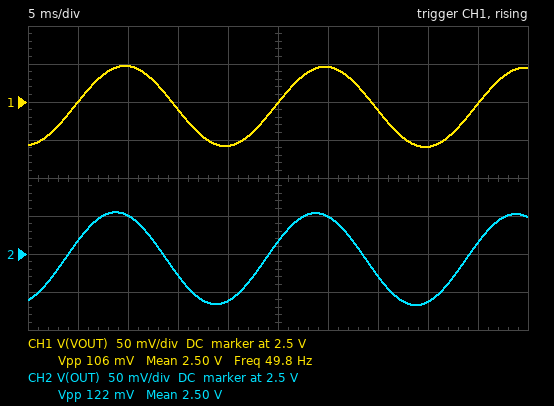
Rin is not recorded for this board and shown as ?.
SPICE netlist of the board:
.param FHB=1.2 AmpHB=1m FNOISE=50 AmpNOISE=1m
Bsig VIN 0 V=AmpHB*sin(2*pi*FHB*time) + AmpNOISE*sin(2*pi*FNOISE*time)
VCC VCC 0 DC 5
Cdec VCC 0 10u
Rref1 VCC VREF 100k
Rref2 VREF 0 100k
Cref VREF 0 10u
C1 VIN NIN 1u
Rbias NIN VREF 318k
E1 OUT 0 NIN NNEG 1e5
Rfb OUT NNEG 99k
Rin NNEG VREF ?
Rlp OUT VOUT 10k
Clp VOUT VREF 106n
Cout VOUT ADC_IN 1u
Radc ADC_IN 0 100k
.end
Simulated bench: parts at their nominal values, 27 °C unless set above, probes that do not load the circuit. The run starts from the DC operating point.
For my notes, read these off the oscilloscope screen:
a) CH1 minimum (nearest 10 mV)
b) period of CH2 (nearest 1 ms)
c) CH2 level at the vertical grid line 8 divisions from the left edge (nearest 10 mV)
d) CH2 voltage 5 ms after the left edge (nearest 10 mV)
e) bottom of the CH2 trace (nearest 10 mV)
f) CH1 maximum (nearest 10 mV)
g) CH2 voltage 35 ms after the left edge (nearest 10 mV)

2.44 V
20 ms
2.44 V
2.52 V
2.43 V
2.55 V
2.47 V
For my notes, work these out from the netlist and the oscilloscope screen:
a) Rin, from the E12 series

680 Ω
